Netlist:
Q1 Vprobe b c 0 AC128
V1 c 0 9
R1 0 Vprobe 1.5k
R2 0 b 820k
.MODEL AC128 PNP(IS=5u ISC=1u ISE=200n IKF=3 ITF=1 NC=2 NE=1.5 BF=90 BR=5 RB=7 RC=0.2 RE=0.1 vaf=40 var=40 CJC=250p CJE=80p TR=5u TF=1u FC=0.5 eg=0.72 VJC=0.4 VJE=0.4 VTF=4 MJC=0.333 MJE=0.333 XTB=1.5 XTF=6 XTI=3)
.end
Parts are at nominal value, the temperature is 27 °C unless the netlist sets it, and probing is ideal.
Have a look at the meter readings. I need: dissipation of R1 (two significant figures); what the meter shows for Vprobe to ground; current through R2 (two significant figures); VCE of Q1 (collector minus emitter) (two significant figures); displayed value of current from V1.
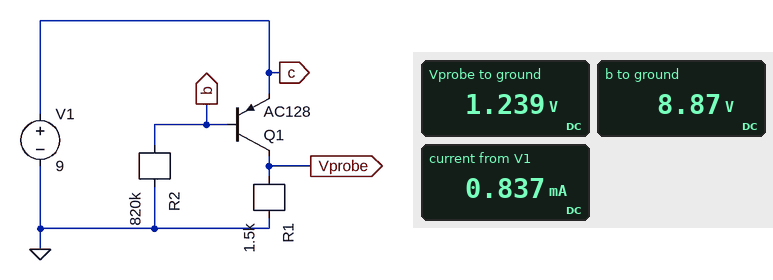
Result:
1.0 mW
1.239 V
11 µA
-7.8 V
0.837 mA
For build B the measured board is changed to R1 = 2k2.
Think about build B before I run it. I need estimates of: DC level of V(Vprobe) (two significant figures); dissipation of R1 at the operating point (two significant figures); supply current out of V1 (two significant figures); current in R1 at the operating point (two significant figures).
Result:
1.8 V
1.5 mW
830 µA
820 µA
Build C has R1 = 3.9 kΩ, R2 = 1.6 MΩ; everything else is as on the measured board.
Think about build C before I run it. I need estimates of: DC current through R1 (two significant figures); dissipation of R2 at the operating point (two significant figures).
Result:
450 µA
49 µW
